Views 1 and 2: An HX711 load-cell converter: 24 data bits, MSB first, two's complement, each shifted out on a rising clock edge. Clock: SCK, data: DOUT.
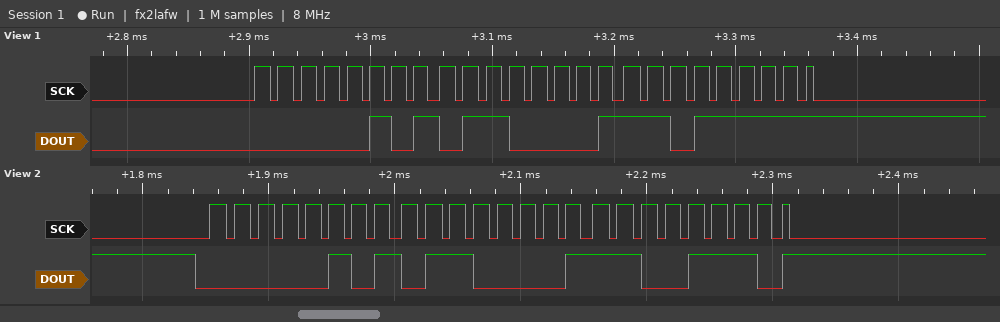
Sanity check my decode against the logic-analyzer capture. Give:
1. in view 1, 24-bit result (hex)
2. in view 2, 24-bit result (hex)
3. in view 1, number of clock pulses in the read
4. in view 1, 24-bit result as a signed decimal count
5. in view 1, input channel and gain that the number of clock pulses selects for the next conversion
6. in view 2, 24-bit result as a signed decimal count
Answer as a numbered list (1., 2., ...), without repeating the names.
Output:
1. 0x0561DF
2. 0x0561CE
3. 25
4. 352735
5. channel A, gain 128
6. 352718
